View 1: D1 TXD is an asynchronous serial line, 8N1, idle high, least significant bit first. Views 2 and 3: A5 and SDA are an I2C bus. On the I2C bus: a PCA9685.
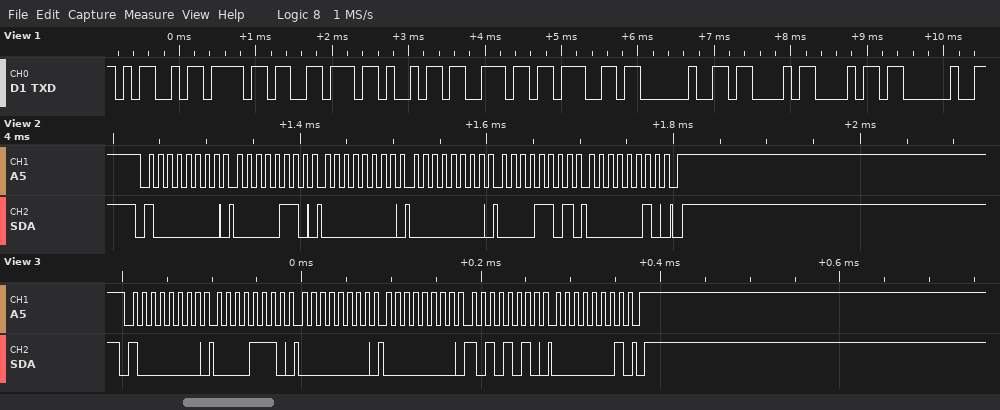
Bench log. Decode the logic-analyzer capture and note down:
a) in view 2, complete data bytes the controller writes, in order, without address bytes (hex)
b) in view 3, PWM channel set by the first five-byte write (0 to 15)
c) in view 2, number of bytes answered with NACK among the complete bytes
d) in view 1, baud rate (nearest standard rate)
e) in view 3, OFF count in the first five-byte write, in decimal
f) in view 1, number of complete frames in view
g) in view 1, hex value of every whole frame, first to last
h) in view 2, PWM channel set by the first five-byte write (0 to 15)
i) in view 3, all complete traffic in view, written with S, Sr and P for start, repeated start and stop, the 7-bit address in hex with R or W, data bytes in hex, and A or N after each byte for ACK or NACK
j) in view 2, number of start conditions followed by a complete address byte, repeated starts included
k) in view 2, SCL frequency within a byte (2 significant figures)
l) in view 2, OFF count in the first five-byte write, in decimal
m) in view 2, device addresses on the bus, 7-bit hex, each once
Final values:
06 00 00 0D 02
2
0
9600 baud
426
10
4D 6F 76 69 6E 67 20 43 68 20
0
S 40W A 0E A 00 A 00 A AA A 01 A P
1
100 kHz
525
0x40
